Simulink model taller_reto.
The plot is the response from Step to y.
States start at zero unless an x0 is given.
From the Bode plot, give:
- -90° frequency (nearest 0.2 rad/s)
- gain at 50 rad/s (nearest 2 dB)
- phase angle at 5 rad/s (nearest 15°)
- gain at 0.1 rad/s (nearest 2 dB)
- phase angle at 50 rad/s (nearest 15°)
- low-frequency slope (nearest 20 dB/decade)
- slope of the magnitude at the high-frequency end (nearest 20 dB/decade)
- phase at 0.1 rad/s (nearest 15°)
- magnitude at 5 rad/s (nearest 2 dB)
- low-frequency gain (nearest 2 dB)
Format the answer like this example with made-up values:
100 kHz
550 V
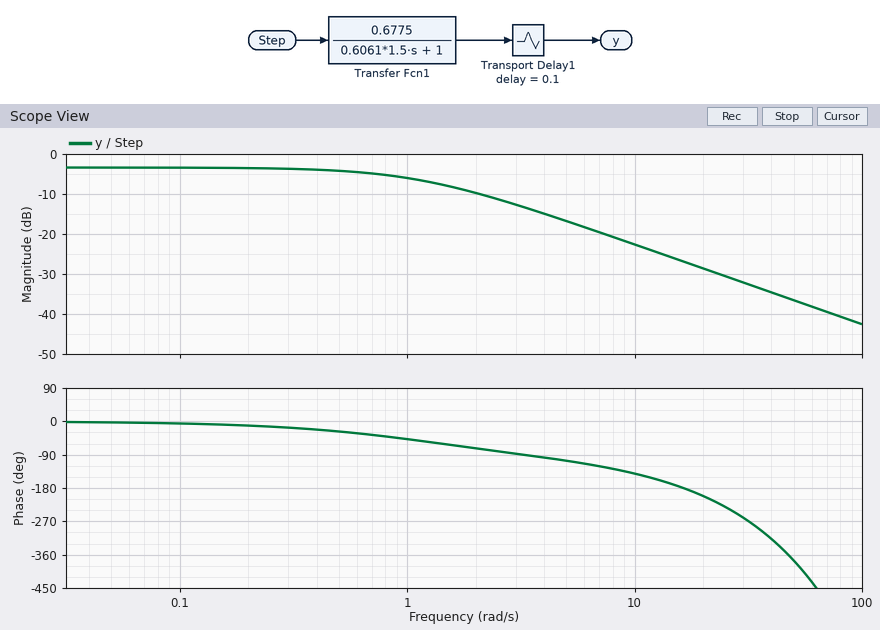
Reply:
3.2 rad/s
-36 dB
-105°
-4 dB
-375°
0 dB/decade
-20 dB/decade
0°
-16 dB
-4 dB
